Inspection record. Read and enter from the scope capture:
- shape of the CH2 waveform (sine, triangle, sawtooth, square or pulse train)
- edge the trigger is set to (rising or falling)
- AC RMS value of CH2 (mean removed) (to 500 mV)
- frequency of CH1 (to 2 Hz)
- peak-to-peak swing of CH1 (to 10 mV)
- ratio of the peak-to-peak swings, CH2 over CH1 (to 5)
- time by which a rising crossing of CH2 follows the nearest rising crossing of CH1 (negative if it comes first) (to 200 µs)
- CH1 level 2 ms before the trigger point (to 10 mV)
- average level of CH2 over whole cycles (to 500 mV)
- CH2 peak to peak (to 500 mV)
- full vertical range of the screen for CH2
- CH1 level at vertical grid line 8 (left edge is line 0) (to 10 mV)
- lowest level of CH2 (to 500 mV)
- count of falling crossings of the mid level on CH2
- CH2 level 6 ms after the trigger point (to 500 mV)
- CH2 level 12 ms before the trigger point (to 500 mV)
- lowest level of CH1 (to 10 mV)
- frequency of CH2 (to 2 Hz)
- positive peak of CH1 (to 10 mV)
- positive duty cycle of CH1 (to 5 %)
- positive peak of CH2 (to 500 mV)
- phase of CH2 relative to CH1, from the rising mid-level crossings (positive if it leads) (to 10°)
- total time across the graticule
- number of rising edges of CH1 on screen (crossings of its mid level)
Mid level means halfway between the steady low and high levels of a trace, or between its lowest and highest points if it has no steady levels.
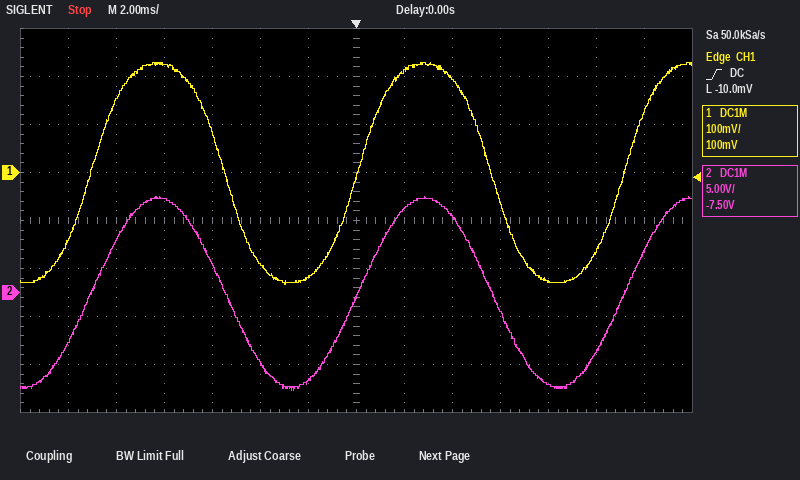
sine
rising
7.0 V
90 Hz
460 mV
45
0.0 ms
-220 mV
0.0 V
20.0 V
40 V
210 mV
-10.0 V
2
-2.0 V
-5.0 V
-230 mV
90 Hz
230 mV
50 %
10.0 V
0°
28 ms
3
